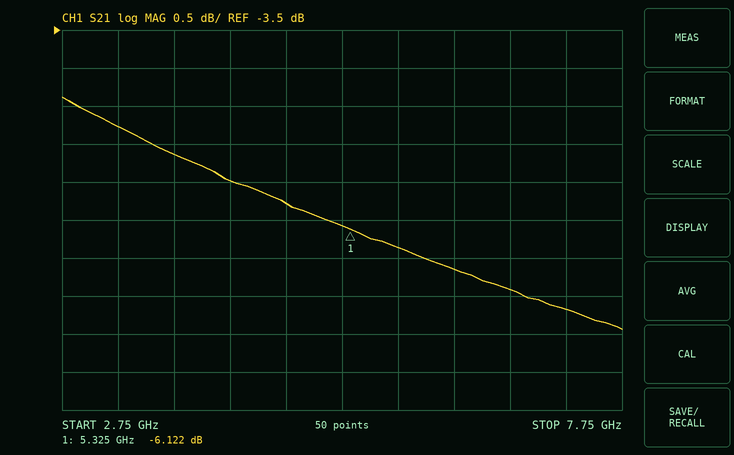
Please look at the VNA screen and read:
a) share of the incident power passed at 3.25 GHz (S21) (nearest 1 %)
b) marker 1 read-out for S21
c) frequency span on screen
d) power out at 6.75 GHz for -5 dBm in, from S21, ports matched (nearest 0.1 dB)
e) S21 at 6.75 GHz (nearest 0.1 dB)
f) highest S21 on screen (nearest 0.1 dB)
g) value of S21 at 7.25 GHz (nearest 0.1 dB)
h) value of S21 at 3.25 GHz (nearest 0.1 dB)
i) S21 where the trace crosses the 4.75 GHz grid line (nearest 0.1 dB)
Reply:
33 %
-6.122 dB
5 GHz
-11.9 dBm
-6.9 dB
-4.4 dB
-7.2 dB
-4.8 dB
-5.8 dB
